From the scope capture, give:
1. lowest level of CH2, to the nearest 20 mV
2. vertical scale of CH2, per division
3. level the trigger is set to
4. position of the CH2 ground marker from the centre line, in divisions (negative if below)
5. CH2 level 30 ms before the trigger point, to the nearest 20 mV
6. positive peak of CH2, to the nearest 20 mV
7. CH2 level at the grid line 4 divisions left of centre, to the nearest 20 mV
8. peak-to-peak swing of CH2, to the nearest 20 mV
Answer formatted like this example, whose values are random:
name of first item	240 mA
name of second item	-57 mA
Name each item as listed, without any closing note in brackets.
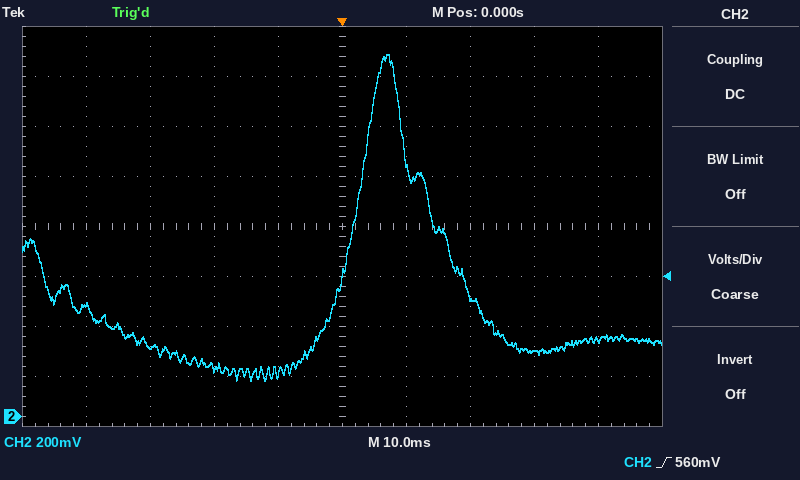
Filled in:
lowest level of CH2, to the nearest 20 mV	140 mV
vertical scale of CH2, per division	200 mV
level the trigger is set to	560 mV
position of the CH2 ground marker from the centre line, in divisions	-3.8 div
CH2 level 30 ms before the trigger point, to the nearest 20 mV	280 mV
positive peak of CH2, to the nearest 20 mV	1.44 V
CH2 level at the grid line 4 divisions left of centre, to the nearest 20 mV	440 mV
peak-to-peak swing of CH2, to the nearest 20 mV	1.30 V
